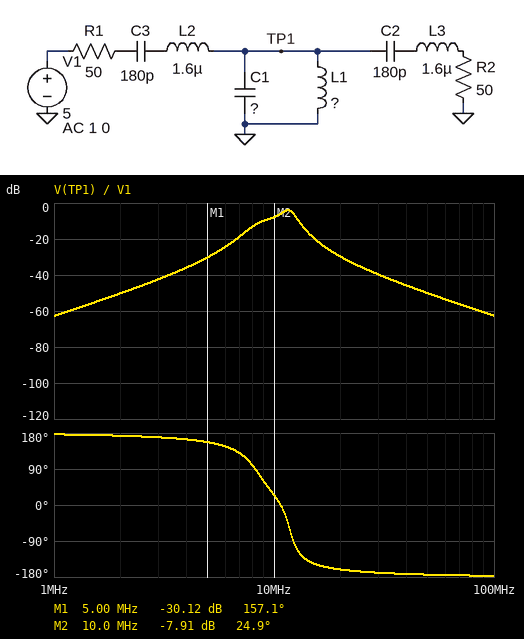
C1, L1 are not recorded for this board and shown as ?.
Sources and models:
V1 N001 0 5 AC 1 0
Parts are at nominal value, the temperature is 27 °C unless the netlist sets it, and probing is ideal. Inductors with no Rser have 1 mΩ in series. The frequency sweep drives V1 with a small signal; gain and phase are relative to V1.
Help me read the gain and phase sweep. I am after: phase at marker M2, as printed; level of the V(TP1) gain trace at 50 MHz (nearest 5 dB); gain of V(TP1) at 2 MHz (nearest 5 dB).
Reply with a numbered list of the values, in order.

1. 24.9 deg
2. -50 dB
3. -50 dB
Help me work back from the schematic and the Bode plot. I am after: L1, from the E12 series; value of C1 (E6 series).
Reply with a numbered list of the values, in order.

1. 100 nH
2. 2.2 nF
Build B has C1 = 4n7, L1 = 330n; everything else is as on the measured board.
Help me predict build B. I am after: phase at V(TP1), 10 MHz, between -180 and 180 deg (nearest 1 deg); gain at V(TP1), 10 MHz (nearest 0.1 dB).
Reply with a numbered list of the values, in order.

1. -95 deg
2. -21.9 dB
